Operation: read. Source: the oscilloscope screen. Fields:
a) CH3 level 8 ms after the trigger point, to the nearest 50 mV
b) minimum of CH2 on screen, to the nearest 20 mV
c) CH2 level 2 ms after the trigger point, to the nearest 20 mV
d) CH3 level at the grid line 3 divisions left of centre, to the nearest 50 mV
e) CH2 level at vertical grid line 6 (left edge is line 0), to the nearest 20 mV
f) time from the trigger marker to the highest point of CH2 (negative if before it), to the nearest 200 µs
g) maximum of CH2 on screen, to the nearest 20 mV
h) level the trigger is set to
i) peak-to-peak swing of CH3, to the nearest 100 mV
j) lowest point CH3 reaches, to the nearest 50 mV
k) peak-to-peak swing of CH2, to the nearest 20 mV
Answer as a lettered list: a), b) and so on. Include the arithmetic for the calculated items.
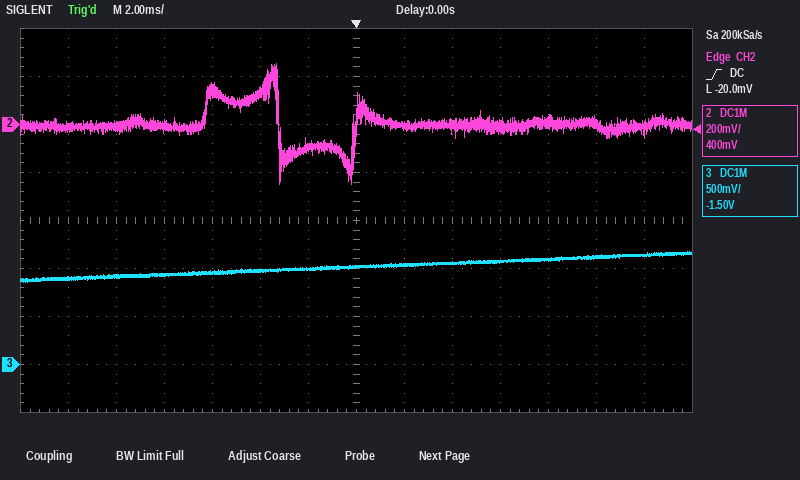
a) 1.10 V
b) -240 mV
c) 0 mV
d) 950 mV
e) -100 mV
f) -3.4 ms
g) 260 mV
h) -20.0 mV
i) 300 mV
j) 850 mV
k) 260 mV − (-240 mV) = 500 mV
